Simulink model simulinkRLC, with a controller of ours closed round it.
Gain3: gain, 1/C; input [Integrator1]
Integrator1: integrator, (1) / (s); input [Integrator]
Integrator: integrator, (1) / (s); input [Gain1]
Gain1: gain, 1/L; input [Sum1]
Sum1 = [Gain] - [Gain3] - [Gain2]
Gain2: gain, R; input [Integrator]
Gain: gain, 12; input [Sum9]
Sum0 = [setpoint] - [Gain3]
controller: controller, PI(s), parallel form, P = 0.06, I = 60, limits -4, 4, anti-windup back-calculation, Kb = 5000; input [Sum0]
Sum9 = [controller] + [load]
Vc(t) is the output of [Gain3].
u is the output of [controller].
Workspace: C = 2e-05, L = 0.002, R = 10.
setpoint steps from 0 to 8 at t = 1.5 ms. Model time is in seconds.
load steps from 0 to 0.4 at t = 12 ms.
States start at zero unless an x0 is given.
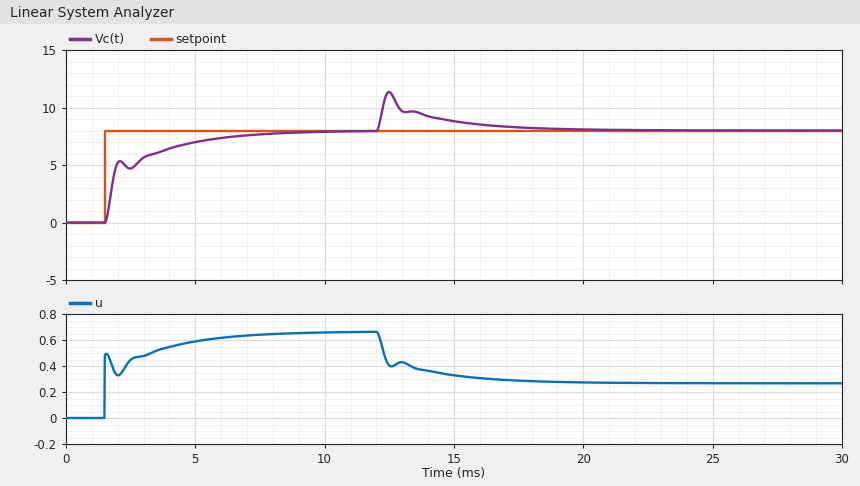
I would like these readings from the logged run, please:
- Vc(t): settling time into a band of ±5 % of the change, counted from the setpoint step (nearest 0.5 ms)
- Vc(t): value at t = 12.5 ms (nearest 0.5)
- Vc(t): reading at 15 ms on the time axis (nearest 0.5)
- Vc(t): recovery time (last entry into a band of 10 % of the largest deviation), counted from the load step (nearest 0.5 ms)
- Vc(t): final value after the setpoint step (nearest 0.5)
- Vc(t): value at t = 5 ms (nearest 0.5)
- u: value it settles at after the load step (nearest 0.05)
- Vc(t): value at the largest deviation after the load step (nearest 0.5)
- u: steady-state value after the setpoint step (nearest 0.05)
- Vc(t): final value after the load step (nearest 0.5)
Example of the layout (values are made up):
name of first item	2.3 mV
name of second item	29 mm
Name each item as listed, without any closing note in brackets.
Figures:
Vc(t): settling time into a band of ±5 % of the change, counted from the setpoint step	5.5 ms
Vc(t): value at t = 12.5 ms	11.5
Vc(t): reading at 15 ms on the time axis	9.0
Vc(t): recovery time (last entry into a band of 10 % of the largest deviation), counted from the load step	5.0 ms
Vc(t): final value after the setpoint step	8.0
Vc(t): value at t = 5 ms	7.0
u: value it settles at after the load step	0.25
Vc(t): value at the largest deviation after the load step	11.5
u: steady-state value after the setpoint step	0.65
Vc(t): final value after the load step	8.0
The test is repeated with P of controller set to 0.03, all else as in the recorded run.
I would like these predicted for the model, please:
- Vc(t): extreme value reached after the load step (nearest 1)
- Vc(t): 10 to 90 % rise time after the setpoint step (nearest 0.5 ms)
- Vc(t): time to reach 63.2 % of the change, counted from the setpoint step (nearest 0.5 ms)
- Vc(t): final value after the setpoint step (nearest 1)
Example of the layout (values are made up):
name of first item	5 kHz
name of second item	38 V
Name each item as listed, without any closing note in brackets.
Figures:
Vc(t): extreme value reached after the load step	12
Vc(t): 10 to 90 % rise time after the setpoint step	3.5 ms
Vc(t): time to reach 63.2 % of the change, counted from the setpoint step	1.5 ms
Vc(t): final value after the setpoint step	8
